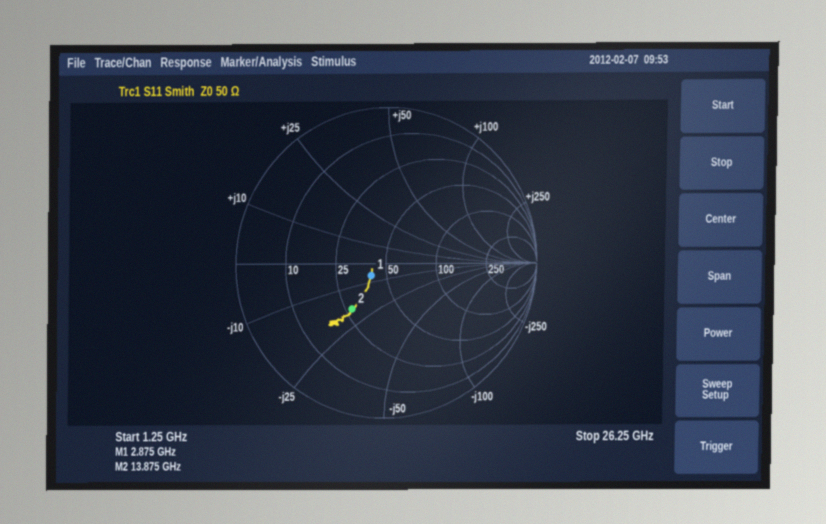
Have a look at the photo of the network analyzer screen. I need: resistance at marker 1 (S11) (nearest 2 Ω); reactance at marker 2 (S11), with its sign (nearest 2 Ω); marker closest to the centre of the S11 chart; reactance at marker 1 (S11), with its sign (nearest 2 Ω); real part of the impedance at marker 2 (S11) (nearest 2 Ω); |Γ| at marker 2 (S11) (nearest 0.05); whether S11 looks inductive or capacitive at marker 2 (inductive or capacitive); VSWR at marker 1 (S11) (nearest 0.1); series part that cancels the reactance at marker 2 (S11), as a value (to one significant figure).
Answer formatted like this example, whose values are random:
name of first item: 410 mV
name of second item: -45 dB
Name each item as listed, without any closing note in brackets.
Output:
resistance at marker 1 (S11): 40 Ω
reactance at marker 2 (S11), with its sign: -18 Ω
marker closest to the centre of the S11 chart: marker 1
reactance at marker 1 (S11), with its sign: -6 Ω
real part of the impedance at marker 2 (S11): 28 Ω
|Γ| at marker 2 (S11): 0.35
whether S11 looks inductive or capacitive at marker 2: capacitive
VSWR at marker 1 (S11): 1.3
series part that cancels the reactance at marker 2 (S11), as a value: 200 pH
